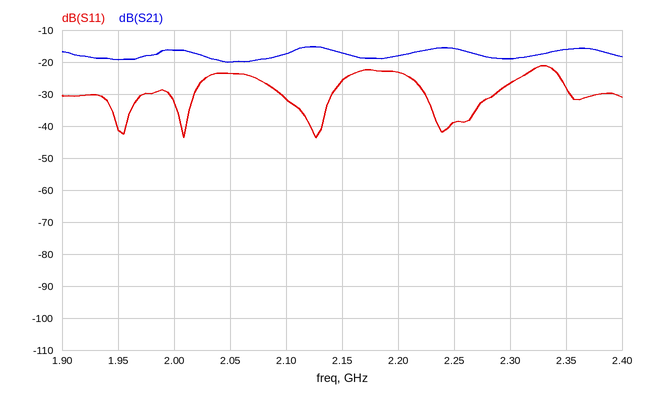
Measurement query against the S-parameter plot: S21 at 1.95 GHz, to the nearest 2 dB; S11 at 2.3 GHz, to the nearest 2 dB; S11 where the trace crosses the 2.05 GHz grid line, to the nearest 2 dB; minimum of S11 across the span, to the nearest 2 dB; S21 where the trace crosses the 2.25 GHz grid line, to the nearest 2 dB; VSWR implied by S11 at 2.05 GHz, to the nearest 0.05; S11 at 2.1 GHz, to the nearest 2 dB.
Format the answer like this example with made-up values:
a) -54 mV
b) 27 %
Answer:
a) -20 dB
b) -26 dB
c) -24 dB
d) -44 dB
e) -16 dB
f) 1.15
g) -32 dB
